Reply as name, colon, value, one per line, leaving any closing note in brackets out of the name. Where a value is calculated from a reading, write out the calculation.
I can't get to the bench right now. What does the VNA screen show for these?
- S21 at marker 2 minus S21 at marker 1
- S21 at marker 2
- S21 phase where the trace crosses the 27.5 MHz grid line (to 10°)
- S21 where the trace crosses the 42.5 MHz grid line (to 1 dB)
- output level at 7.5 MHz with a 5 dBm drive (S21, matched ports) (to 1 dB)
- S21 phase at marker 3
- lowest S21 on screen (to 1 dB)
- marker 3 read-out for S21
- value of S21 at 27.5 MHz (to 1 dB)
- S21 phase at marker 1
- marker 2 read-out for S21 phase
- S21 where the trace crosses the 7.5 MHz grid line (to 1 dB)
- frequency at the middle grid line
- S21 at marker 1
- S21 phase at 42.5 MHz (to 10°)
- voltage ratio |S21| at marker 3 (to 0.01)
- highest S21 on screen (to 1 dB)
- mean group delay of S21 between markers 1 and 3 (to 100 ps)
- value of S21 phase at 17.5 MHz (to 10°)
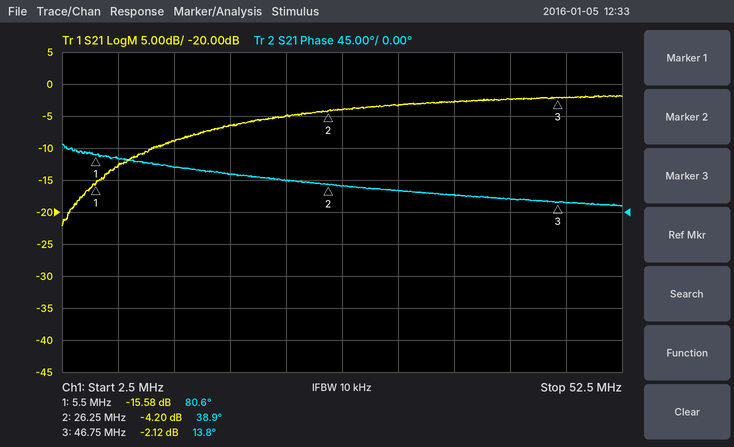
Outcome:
S21 at marker 2 minus S21 at marker 1: -4.2 − (-15.58) = 11.38 dB
S21 at marker 2: -4.20 dB
S21 phase where the trace crosses the 27.5 MHz grid line: 40°
S21 where the trace crosses the 42.5 MHz grid line: -2 dB
output level at 7.5 MHz with a 5 dBm drive (S21, matched ports): 5 dBm + (-13 dB) = -8 dBm
S21 phase at marker 3: 13.8°
lowest S21 on screen: -22 dB
marker 3 read-out for S21: -2.12 dB
value of S21 at 27.5 MHz: -4 dB
S21 phase at marker 1: 80.6°
marker 2 read-out for S21 phase: 38.9°
S21 where the trace crosses the 7.5 MHz grid line: -13 dB
frequency at the middle grid line: 27.5 MHz
S21 at marker 1: -15.58 dB
S21 phase at 42.5 MHz: 20°
voltage ratio |S21| at marker 3: 10^(-2.12/20) ≈ 0.78
highest S21 on screen: -2 dB
mean group delay of S21 between markers 1 and 3: −(13.8° − (80.6°))/(360° × 41.25 MHz) ≈ 4.5 ns
value of S21 phase at 17.5 MHz: 50°
